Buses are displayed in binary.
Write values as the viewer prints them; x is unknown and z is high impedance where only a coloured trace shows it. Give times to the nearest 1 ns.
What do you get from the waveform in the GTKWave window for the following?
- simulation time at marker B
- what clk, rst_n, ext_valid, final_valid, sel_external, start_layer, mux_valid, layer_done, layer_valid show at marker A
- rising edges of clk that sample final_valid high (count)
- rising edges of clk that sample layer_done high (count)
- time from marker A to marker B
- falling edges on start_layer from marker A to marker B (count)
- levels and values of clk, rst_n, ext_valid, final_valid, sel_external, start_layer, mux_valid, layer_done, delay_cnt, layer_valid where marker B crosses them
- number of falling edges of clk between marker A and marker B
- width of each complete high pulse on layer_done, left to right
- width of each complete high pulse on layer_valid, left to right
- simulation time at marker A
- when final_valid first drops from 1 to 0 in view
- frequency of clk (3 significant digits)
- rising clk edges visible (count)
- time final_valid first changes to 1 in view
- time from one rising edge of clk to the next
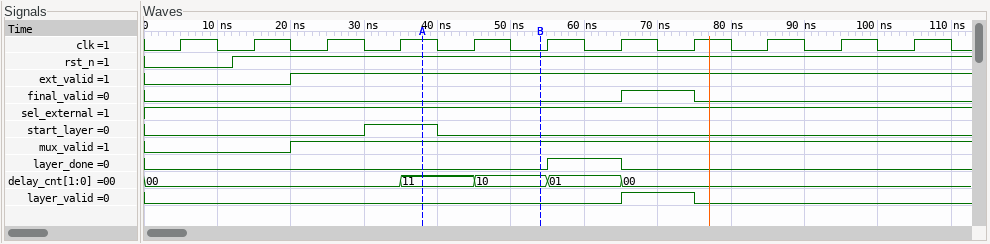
54 ns
clk=1, rst_n=1, ext_valid=1, final_valid=0, sel_external=1, start_layer=1, mux_valid=1, layer_done=0, layer_valid=0
1
1
16 ns
1
clk=0, rst_n=1, ext_valid=1, final_valid=0, sel_external=1, start_layer=0, mux_valid=1, layer_done=0, delay_cnt=10, layer_valid=0
2
10 ns
10 ns
38 ns
75 ns
100 MHz
11
65 ns
10 ns
